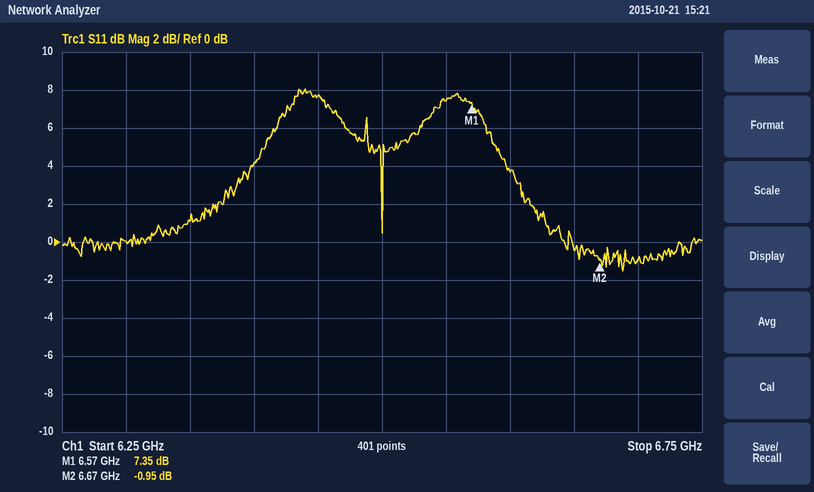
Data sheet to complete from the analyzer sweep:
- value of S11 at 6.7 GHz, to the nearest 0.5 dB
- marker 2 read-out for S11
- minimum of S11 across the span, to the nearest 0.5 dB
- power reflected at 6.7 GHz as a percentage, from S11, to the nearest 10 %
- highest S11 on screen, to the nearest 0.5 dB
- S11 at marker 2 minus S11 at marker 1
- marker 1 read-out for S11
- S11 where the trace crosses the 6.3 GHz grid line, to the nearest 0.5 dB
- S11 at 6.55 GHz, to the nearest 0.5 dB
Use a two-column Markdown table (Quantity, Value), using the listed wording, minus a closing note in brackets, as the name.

| Quantity | Value |
|---|---|
| value of S11 at 6.7 GHz, to the nearest 0.5 dB | -1.0 dB |
| marker 2 read-out for S11 | -0.95 dB |
| minimum of S11 across the span, to the nearest 0.5 dB | -1.5 dB |
| power reflected at 6.7 GHz as a percentage, from S11, to the nearest 10 % | 80 % |
| highest S11 on screen, to the nearest 0.5 dB | 8.0 dB |
| S11 at marker 2 minus S11 at marker 1 | -8.30 dB |
| marker 1 read-out for S11 | 7.35 dB |
| S11 where the trace crosses the 6.3 GHz grid line, to the nearest 0.5 dB | 0.0 dB |
| S11 at 6.55 GHz, to the nearest 0.5 dB | 7.5 dB |
